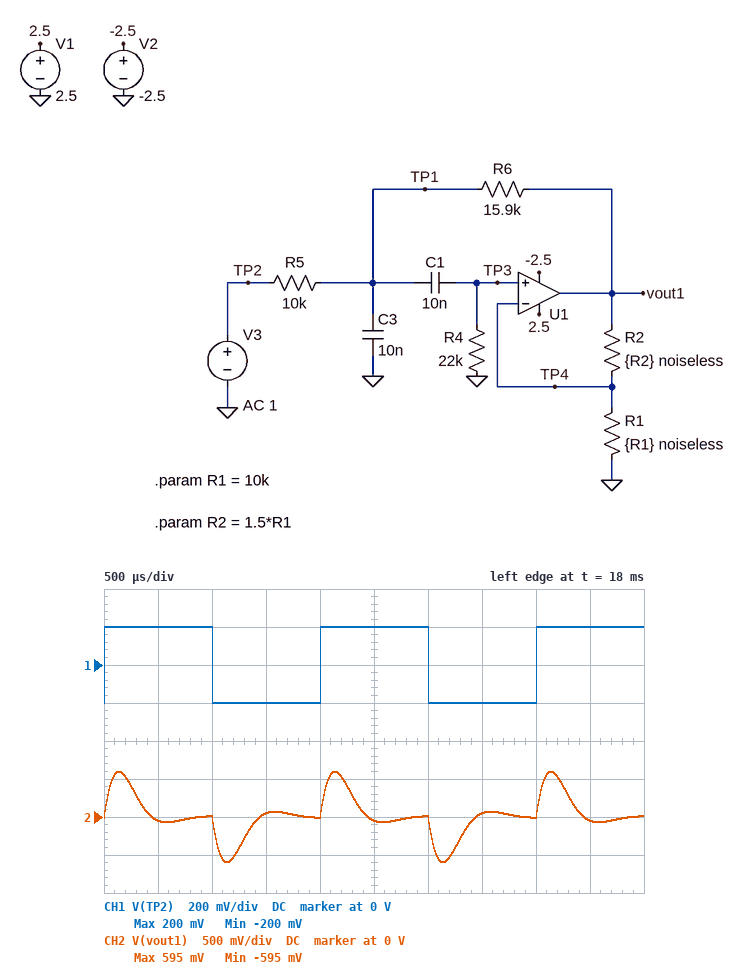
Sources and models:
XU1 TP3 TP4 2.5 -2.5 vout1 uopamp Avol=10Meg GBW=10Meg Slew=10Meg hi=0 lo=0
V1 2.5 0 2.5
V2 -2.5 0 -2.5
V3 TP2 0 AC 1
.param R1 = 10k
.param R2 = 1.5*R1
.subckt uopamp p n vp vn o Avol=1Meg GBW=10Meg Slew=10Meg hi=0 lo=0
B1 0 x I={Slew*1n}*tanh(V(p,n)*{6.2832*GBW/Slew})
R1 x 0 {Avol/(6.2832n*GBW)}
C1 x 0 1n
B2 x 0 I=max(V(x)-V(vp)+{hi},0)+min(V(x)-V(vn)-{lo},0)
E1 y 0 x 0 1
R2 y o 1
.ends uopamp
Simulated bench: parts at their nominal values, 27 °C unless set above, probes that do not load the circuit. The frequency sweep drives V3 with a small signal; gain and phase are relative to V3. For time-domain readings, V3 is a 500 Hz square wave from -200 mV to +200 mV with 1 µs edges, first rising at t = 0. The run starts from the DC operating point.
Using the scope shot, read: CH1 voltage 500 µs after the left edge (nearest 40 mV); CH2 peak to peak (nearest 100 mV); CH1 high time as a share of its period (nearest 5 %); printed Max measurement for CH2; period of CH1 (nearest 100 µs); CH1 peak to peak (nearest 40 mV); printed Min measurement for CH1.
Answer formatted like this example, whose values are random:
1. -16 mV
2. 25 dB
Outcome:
1. 200 mV
2. 1.2 V
3. 50 %
4. 595 mV
5. 2.0 ms
6. 400 mV
7. -200 mV
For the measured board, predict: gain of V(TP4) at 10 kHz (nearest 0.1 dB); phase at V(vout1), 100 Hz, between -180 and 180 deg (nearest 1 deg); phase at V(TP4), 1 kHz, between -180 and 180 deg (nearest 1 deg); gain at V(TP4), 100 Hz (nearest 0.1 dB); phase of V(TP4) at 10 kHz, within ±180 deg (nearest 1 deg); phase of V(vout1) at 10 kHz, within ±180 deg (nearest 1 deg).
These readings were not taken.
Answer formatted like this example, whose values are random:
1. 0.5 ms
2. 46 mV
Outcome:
1. -15.9 dB
2. 85 deg
3. 30 deg
4. -21.4 dB
5. -81 deg
6. -81 deg
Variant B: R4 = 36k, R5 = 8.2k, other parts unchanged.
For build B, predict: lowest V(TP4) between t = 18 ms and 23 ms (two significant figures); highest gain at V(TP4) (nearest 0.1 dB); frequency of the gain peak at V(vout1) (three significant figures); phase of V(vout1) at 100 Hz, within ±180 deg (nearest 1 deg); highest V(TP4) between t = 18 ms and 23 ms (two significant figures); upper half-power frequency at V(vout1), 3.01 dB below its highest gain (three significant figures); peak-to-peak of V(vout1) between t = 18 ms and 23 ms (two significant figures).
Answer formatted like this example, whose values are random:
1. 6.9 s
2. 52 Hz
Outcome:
1. -340 mV
2. 3.3 dB
3. 1.14 kHz
4. 84 deg
5. 340 mV
6. 1.98 kHz
7. 1.7 V
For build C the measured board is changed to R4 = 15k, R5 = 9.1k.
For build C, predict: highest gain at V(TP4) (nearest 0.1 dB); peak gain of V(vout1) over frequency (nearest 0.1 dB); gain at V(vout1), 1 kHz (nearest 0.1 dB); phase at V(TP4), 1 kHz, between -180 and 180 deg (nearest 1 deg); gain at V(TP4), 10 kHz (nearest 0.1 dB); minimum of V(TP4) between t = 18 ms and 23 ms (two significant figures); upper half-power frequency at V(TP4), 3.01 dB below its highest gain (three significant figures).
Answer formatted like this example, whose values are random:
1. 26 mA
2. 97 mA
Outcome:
1. -2.6 dB
2. 5.3 dB
3. 3.1 dB
4. 39 deg
5. -15.1 dB
6. -190 mV
7. 3.26 kHz
